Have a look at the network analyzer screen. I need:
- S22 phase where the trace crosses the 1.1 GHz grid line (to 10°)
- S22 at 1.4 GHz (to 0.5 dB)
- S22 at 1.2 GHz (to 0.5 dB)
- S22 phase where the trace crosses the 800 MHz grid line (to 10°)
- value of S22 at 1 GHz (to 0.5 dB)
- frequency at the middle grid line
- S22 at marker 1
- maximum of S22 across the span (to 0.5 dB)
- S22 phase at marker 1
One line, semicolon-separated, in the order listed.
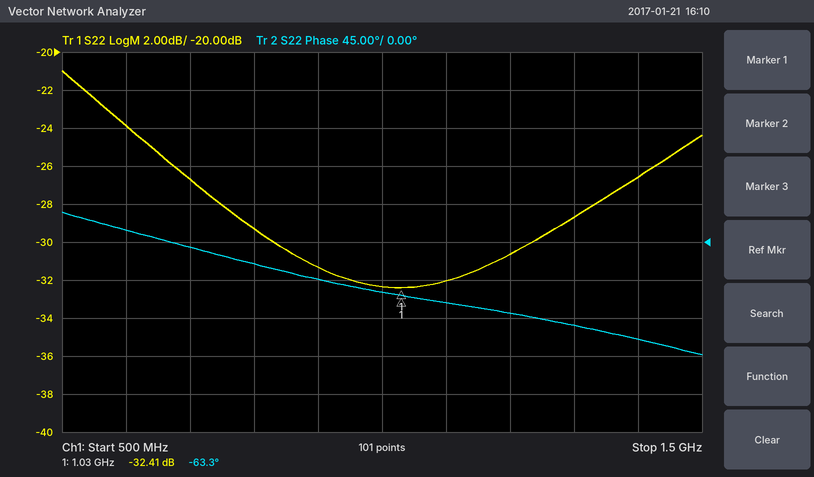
-70°; -26.5 dB; -30.5 dB; -30°; -32.5 dB; 1 GHz; -32.41 dB; -21.0 dB; -63.3°
